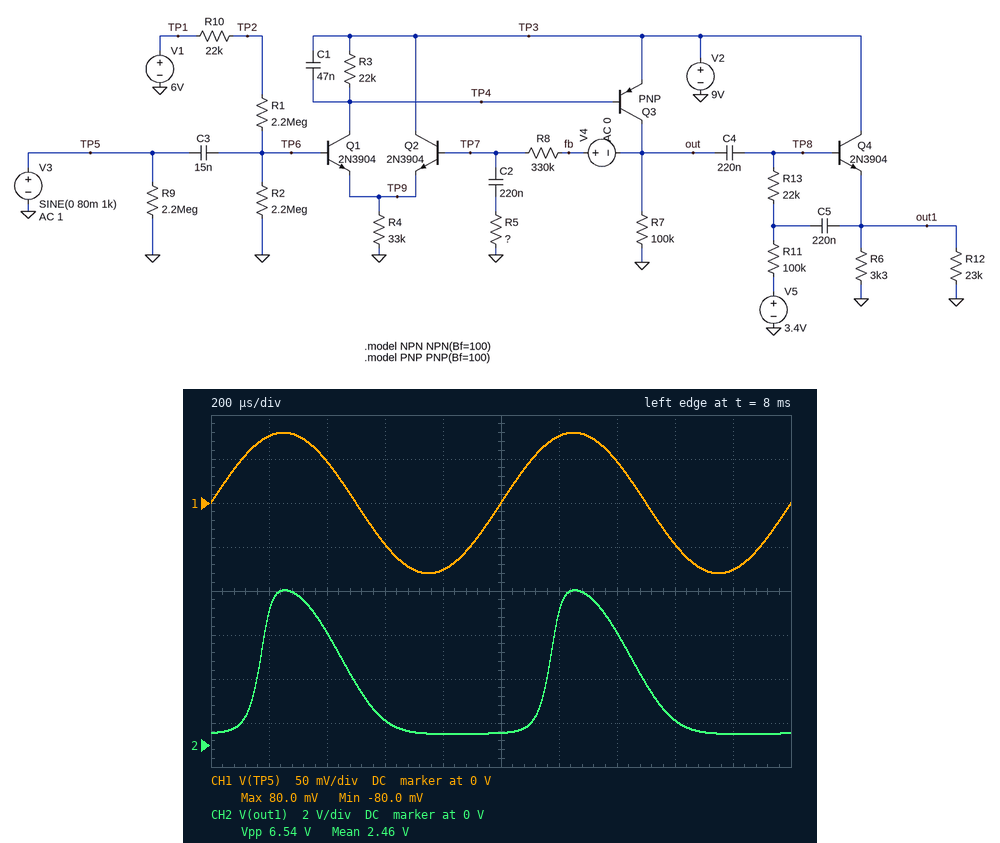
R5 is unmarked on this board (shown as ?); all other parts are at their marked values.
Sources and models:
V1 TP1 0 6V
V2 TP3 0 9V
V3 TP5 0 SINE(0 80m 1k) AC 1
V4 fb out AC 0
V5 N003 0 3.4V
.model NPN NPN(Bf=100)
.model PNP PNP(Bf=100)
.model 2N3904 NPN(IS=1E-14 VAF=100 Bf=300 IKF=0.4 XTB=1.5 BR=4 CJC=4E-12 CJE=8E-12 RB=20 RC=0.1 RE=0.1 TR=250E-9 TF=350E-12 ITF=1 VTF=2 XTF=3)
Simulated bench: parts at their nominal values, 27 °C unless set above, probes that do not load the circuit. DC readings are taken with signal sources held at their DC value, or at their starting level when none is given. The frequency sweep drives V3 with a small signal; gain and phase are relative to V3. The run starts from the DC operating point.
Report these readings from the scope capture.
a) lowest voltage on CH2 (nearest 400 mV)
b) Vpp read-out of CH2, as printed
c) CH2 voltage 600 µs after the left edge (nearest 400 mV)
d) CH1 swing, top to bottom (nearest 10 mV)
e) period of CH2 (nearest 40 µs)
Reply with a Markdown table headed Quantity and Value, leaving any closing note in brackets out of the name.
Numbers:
| Quantity | Value |
|---|---|
| lowest voltage on CH2 | 400 mV |
| Vpp read-out of CH2, as printed | 6.54 V |
| CH2 voltage 600 µs after the left edge | 1.2 V |
| CH1 swing, top to bottom | 160 mV |
| period of CH2 | 1.00 ms |
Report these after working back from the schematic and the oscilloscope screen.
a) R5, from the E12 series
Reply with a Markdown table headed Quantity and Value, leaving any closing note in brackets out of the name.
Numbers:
| Quantity | Value |
|---|---|
| R5, from the E12 series | 5.6 kΩ |
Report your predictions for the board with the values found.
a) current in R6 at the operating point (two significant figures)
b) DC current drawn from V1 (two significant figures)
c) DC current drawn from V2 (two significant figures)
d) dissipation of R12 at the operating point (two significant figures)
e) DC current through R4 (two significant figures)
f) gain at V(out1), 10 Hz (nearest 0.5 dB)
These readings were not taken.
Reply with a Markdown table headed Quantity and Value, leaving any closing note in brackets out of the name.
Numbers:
| Quantity | Value |
|---|---|
| current in R6 at the operating point | 740 µA |
| DC current drawn from V1 | 1.4 µA |
| DC current drawn from V2 | 940 µA |
| dissipation of R12 at the operating point | 260 µW |
| DC current through R4 | 70 µA |
| gain at V(out1), 10 Hz | 10.0 dB |
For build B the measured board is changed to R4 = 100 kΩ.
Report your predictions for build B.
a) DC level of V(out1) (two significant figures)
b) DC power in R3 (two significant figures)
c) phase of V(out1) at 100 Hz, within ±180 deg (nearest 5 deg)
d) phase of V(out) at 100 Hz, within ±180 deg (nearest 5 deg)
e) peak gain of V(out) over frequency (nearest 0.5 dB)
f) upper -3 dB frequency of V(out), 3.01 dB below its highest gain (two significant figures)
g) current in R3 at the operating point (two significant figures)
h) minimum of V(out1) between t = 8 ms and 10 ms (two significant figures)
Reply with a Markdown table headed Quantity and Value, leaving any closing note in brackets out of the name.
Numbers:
| Quantity | Value |
|---|---|
| DC level of V(out1) | 2.4 V |
| DC power in R3 | 12 µW |
| phase of V(out1) at 100 Hz, within ±180 deg | -15 deg |
| phase of V(out) at 100 Hz, within ±180 deg | -20 deg |
| peak gain of V(out) over frequency | -30.5 dB |
| upper -3 dB frequency of V(out), 3.01 dB below its highest gain | 5.5 MHz |
| current in R3 at the operating point | 23 µA |
| minimum of V(out1) between t = 8 ms and 10 ms | 2.4 V |
